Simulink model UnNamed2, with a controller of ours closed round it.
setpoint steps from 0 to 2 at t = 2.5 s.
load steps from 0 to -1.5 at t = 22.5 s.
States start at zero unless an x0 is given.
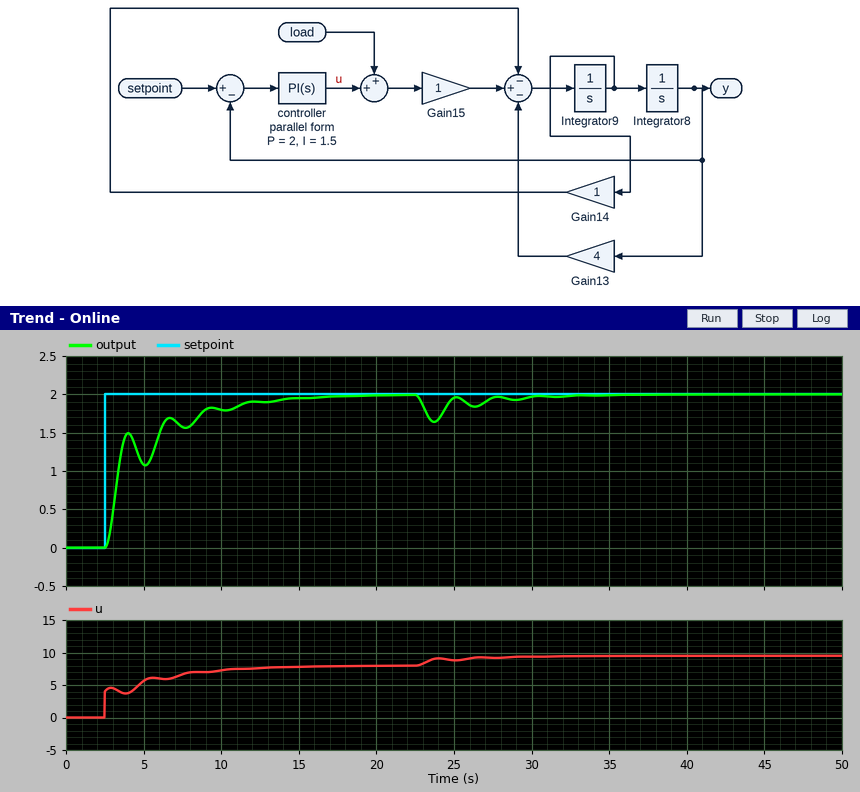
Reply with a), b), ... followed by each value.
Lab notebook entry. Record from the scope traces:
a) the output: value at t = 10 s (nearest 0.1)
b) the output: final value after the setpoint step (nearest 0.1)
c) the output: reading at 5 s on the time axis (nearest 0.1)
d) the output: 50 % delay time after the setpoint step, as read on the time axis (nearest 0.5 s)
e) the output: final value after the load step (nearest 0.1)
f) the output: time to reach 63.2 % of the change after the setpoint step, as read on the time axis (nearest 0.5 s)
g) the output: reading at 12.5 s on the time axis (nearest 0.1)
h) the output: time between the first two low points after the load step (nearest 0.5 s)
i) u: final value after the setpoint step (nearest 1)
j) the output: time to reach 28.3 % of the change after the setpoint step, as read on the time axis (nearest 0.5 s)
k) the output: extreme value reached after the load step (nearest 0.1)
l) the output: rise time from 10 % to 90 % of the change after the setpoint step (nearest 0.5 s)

a) 1.8
b) 2.0
c) 1.1
d) 3.5 s
e) 2.0
f) 3.5 s
g) 1.9
h) 2.5 s
i) 8
j) 3.0 s
k) 1.6
l) 6.0 s
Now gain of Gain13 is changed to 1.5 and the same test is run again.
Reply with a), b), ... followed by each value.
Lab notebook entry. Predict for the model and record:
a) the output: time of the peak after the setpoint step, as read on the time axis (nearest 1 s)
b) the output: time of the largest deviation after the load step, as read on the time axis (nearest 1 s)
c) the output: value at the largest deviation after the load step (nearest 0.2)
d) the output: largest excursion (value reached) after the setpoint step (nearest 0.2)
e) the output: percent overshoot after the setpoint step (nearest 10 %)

a) 4 s
b) 24 s
c) 1.4
d) 2.4
e) 20 %
